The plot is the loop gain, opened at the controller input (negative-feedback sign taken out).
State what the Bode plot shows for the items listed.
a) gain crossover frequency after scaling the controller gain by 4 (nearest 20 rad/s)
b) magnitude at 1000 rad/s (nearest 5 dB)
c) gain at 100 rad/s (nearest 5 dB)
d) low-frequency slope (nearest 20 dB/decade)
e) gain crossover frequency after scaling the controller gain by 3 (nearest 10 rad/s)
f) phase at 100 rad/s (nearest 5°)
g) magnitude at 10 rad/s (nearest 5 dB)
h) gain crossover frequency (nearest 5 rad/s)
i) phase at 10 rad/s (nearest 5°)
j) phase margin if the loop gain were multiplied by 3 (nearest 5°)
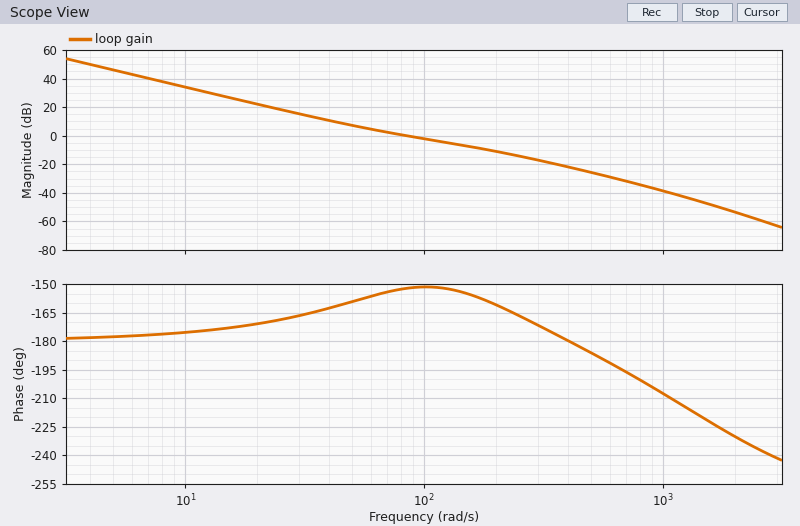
220 rad/s
-40 dB
0 dB
-40 dB/decade
180 rad/s
-150°
35 dB
85 rad/s
-175°
20°
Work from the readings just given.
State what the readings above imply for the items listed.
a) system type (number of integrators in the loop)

2
